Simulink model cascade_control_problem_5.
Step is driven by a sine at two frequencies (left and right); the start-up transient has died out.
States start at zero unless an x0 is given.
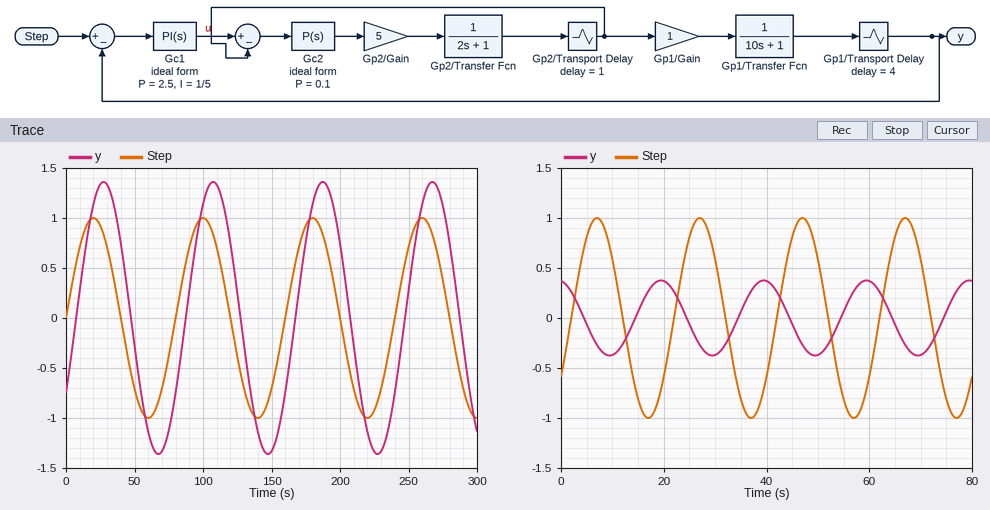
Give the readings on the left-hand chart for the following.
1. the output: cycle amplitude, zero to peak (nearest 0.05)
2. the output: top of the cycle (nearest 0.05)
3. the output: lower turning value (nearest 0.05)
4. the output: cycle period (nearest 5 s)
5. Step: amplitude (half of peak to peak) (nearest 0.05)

1.35
1.35
-1.35
80 s
1.00
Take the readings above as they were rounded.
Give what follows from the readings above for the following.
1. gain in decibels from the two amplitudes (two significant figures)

2.6 dB
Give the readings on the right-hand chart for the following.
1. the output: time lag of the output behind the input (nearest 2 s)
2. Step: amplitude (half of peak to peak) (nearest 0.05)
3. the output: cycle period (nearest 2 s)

12 s
1.00
20 s
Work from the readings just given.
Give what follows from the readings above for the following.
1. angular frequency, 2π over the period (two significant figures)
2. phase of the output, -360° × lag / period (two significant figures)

0.31 rad/s
-220°
